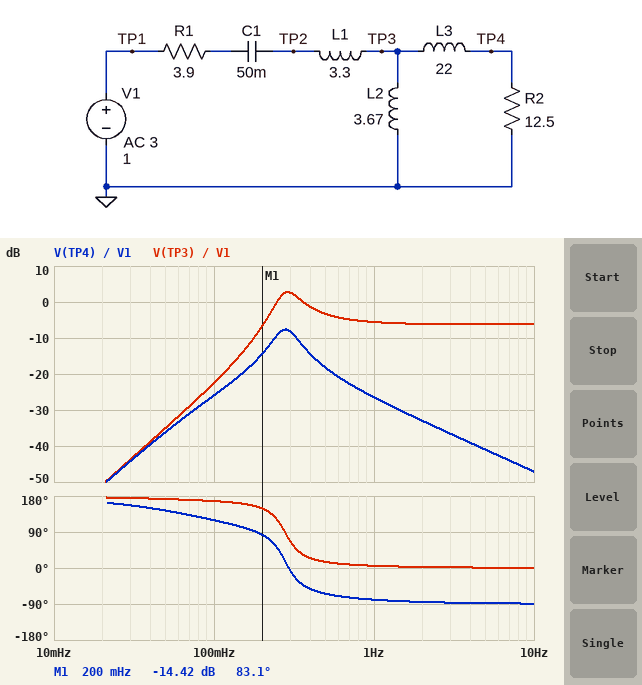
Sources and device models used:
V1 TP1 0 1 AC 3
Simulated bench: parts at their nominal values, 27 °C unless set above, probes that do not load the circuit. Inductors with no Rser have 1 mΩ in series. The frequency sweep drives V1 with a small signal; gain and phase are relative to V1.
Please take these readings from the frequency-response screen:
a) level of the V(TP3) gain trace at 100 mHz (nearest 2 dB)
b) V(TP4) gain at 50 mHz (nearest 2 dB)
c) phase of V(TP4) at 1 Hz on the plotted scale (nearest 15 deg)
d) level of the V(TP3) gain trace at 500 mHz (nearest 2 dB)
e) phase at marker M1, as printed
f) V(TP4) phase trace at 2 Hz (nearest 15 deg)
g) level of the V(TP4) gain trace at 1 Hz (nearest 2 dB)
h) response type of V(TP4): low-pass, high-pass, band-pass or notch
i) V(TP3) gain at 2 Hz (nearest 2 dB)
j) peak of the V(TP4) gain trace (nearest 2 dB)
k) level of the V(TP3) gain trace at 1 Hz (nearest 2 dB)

-22 dB
-36 dB
-75 deg
-4 dB
83.1 deg
-90 deg
-26 dB
band-pass
-6 dB
-8 dB
-6 dB
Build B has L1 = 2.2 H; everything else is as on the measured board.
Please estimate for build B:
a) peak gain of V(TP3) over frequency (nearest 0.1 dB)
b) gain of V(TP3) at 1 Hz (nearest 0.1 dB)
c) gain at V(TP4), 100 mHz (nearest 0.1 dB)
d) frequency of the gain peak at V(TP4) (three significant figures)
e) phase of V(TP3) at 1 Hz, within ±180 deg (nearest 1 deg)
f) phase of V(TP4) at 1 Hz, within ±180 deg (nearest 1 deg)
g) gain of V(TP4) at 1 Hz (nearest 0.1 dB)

3.6 dB
-3.8 dB
-26.1 dB
308 mHz
7 deg
-78 deg
-24.7 dB
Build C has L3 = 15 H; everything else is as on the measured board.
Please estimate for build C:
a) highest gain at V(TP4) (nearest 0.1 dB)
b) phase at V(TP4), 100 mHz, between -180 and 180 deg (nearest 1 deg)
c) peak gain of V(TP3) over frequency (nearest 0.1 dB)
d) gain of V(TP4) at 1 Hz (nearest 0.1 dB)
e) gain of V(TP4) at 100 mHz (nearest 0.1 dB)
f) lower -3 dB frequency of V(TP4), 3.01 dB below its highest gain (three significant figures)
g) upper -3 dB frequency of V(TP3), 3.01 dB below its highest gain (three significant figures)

-5.5 dB
128 deg
2.1 dB
-23.5 dB
-24.4 dB
235 mHz
381 mHz
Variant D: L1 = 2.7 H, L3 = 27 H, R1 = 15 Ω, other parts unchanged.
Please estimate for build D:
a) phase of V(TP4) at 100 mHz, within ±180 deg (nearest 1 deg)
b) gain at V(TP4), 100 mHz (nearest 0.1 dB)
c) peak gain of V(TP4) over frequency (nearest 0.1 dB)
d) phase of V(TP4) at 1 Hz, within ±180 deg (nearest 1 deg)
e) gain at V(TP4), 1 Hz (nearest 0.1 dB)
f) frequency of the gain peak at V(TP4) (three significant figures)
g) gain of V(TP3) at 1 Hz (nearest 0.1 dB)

95 deg
-28.1 dB
-20.3 dB
-62 deg
-28.0 dB
298 mHz
-5.3 dB
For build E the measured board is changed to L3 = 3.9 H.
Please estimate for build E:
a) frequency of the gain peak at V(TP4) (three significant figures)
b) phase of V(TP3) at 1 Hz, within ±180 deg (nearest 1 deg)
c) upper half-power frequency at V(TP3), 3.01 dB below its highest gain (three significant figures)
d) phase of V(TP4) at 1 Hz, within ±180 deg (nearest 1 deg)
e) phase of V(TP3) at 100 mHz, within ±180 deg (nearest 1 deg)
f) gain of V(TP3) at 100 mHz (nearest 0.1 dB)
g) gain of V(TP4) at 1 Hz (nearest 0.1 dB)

295 mHz
0 deg
437 mHz
-63 deg
161 deg
-22.1 dB
-14.4 dB
